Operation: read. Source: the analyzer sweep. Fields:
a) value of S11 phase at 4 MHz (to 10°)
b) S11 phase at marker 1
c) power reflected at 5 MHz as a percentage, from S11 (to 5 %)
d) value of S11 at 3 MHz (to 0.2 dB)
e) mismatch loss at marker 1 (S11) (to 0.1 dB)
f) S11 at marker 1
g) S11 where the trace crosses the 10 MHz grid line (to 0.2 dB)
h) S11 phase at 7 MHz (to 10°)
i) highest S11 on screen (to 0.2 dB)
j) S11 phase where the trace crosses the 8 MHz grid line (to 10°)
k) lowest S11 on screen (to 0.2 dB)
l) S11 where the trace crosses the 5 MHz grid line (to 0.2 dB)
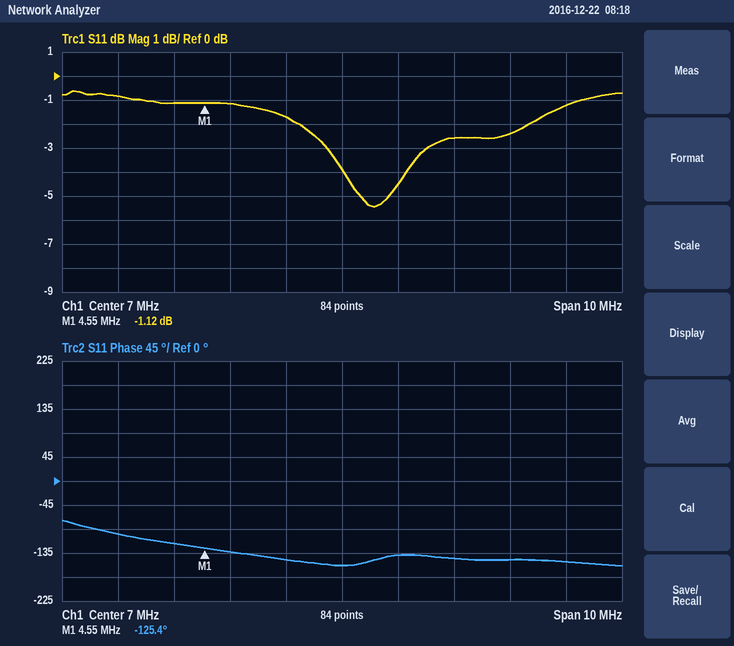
-120°
-125.4°
75 %
-0.8 dB
6.4 dB
-1.12 dB
-2.4 dB
-160°
-0.6 dB
-140°
-5.4 dB
-1.2 dB
